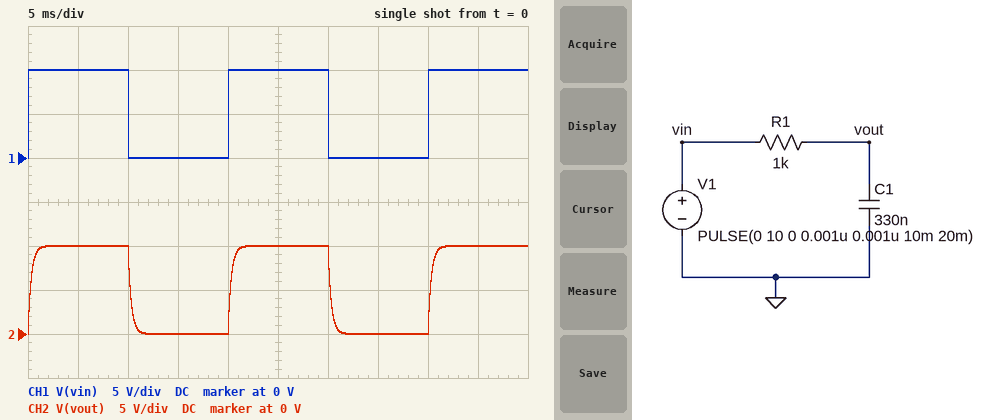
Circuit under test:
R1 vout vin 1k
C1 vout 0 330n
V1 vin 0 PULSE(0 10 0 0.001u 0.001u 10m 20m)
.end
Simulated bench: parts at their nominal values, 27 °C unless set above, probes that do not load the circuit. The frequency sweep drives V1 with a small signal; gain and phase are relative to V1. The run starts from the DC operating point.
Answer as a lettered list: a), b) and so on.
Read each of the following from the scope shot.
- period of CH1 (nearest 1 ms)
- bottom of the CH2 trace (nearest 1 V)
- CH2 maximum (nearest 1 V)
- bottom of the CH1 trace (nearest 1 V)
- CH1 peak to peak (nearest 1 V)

a) 20 ms
b) 0 V
c) 10 V
d) 0 V
e) 10 V
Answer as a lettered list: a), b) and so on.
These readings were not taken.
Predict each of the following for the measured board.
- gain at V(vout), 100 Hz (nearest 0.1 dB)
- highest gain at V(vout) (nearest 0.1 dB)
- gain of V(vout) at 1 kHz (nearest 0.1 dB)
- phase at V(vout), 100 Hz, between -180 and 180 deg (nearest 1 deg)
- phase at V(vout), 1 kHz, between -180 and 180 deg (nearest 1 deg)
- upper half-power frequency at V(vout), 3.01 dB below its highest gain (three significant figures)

a) -0.2 dB
b) 0 dB
c) -7.2 dB
d) -12 deg
e) -64 deg
f) 482 Hz
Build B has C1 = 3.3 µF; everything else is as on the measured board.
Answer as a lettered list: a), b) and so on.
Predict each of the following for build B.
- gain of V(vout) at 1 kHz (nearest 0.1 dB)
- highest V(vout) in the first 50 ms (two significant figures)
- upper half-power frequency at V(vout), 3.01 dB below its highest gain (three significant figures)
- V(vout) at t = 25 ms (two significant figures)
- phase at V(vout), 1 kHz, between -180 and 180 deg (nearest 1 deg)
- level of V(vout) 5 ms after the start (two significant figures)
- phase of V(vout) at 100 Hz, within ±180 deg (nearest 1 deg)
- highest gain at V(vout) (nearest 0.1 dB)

a) -26.3 dB
b) 9.5 V
c) 48.2 Hz
d) 7.9 V
e) -87 deg
f) 7.8 V
g) -64 deg
h) 0 dB
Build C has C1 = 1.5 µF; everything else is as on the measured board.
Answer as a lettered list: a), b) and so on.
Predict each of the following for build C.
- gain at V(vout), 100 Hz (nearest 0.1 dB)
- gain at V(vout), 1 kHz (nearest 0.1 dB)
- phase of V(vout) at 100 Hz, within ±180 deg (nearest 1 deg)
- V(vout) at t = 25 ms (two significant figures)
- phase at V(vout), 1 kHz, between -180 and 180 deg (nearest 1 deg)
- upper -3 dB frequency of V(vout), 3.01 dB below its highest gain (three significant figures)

a) -2.8 dB
b) -19.5 dB
c) -43 deg
d) 9.6 V
e) -84 deg
f) 106 Hz
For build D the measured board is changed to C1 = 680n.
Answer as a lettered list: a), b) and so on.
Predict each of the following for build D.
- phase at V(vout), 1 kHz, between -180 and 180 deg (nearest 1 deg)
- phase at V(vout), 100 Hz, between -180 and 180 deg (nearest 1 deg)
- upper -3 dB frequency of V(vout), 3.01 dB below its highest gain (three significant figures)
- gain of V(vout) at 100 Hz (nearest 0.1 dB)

a) -77 deg
b) -23 deg
c) 234 Hz
d) -0.7 dB
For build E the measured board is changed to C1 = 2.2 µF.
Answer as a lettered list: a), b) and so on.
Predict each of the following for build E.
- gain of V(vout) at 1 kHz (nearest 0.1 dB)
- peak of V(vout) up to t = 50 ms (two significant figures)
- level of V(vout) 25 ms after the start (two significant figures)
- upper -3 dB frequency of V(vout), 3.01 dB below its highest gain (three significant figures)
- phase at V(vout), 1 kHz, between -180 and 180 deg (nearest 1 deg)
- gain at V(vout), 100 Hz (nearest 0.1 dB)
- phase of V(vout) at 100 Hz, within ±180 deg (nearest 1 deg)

a) -22.8 dB
b) 9.9 V
c) 9.0 V
d) 72.3 Hz
e) -86 deg
f) -4.6 dB
g) -54 deg
